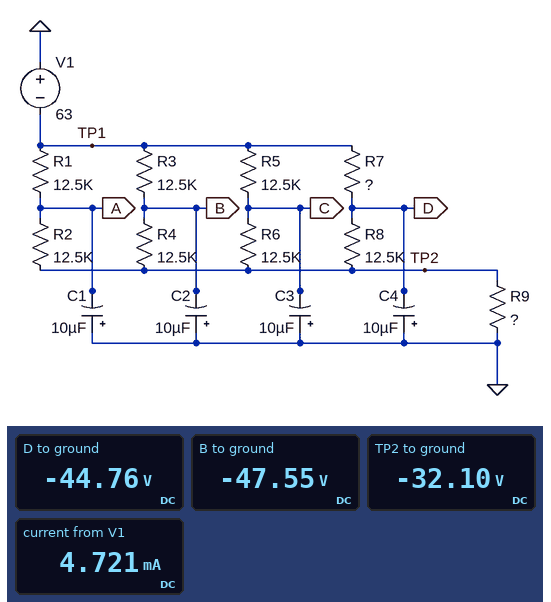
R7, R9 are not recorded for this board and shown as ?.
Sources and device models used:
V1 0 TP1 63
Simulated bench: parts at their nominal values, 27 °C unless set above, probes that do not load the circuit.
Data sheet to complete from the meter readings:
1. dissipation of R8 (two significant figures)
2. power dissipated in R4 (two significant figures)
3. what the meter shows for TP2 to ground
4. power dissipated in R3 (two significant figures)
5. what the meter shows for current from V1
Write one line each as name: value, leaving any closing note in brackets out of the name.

dissipation of R8: 13 mW
power dissipated in R4: 19 mW
what the meter shows for TP2 to ground: -32.10 V
power dissipated in R3: 19 mW
what the meter shows for current from V1: 4.721 mA
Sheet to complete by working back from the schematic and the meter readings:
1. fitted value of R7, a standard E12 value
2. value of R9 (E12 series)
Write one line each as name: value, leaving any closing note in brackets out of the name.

fitted value of R7, a standard E12 value: 18 kΩ
value of R9: 6.8 kΩ
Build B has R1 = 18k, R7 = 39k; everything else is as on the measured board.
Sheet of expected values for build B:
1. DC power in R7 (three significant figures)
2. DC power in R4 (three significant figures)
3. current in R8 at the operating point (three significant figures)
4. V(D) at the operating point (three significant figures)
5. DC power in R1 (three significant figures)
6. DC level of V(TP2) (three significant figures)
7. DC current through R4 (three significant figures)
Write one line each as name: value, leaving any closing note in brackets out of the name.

DC power in R7: 16.2 mW
DC power in R4: 22.0 mW
current in R8 at the operating point: 644 µA
V(D) at the operating point: -37.9 V
DC power in R1: 21.3 mW
DC level of V(TP2): -29.8 V
DC current through R4: 1.33 mA
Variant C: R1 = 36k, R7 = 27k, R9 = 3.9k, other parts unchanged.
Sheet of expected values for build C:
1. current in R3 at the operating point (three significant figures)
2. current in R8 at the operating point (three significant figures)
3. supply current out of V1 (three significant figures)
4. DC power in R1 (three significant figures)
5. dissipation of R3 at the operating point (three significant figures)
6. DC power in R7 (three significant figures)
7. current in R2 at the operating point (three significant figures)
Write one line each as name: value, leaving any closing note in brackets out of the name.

current in R3 at the operating point: 1.69 mA
current in R8 at the operating point: 1.07 mA
supply current out of V1: 5.32 mA
DC power in R1: 27.3 mW
dissipation of R3 at the operating point: 35.7 mW
DC power in R7: 30.9 mW
current in R2 at the operating point: 871 µA
